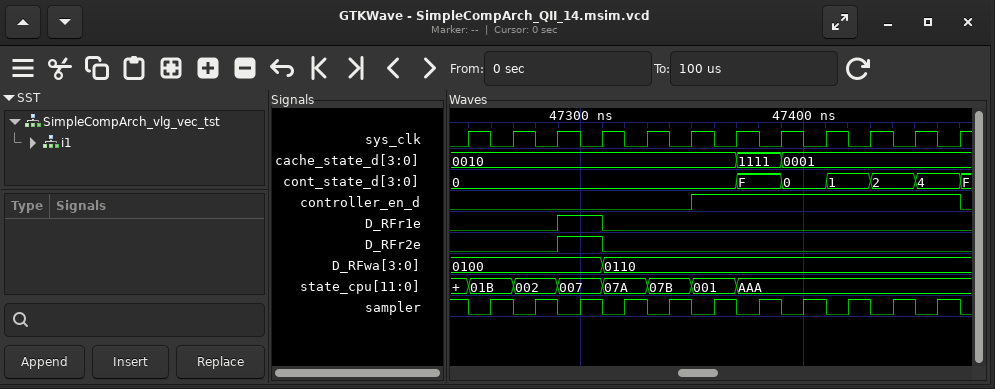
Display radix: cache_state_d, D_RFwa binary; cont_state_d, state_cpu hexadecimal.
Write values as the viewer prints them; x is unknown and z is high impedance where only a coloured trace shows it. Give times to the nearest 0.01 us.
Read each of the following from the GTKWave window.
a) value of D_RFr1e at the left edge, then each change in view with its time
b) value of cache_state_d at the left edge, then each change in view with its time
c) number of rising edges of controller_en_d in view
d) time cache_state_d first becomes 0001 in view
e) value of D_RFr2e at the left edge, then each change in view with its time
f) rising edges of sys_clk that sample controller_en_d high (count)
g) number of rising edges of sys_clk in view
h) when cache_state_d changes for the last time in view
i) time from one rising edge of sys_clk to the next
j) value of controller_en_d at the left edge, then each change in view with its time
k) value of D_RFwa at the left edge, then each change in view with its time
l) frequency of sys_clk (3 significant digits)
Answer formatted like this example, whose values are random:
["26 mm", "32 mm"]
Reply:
["0, 1 at 47.29 us, 0 at 47.31 us", "0010, 1111 at 47.37 us, 0001 at 47.39 us", "1", "47.39 us", "0, 1 at 47.29 us, 0 at 47.31 us", "6", "12", "47.39 us", "0.02 us", "0, 1 at 47.35 us, 0 at 47.47 us", "0100, 0110 at 47.31 us", "50.0 MHz"]
